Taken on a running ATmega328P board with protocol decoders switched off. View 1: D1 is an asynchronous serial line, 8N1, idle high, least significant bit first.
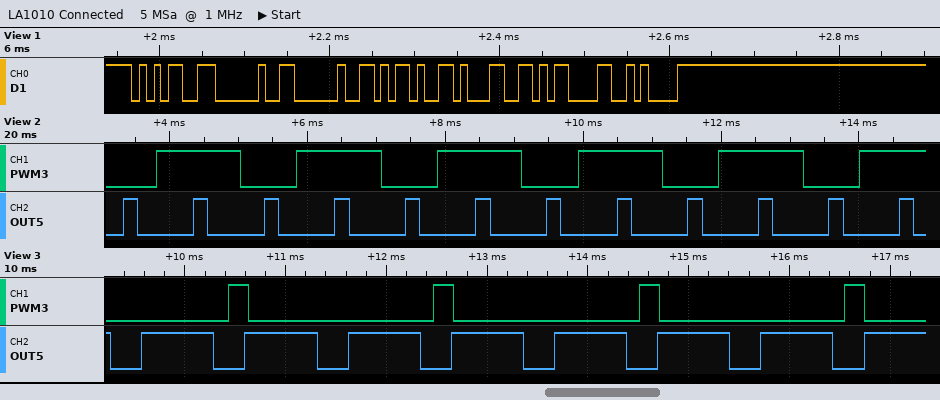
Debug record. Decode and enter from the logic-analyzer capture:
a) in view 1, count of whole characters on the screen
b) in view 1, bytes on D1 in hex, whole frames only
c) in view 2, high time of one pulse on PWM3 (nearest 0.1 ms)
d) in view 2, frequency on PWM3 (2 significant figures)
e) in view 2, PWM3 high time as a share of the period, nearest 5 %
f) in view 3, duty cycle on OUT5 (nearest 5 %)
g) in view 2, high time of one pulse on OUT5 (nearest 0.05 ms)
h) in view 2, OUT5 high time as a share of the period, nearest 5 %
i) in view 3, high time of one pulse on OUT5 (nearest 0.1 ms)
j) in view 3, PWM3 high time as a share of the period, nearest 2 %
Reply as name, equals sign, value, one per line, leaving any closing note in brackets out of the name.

in view 1, count of whole characters on the screen = 7
in view 1, bytes on D1 in hex, whole frames only = 35 20 20 2D 31 0D 0A
in view 2, high time of one pulse on PWM3 = 1.2 ms
in view 2, frequency on PWM3 = 490 Hz
in view 2, PWM3 high time as a share of the period, nearest 5 % = 60 %
in view 3, duty cycle on OUT5 = 70 %
in view 2, high time of one pulse on OUT5 = 0.20 ms
in view 2, OUT5 high time as a share of the period, nearest 5 % = 20 %
in view 3, high time of one pulse on OUT5 = 0.7 ms
in view 3, PWM3 high time as a share of the period, nearest 2 % = 10 %
